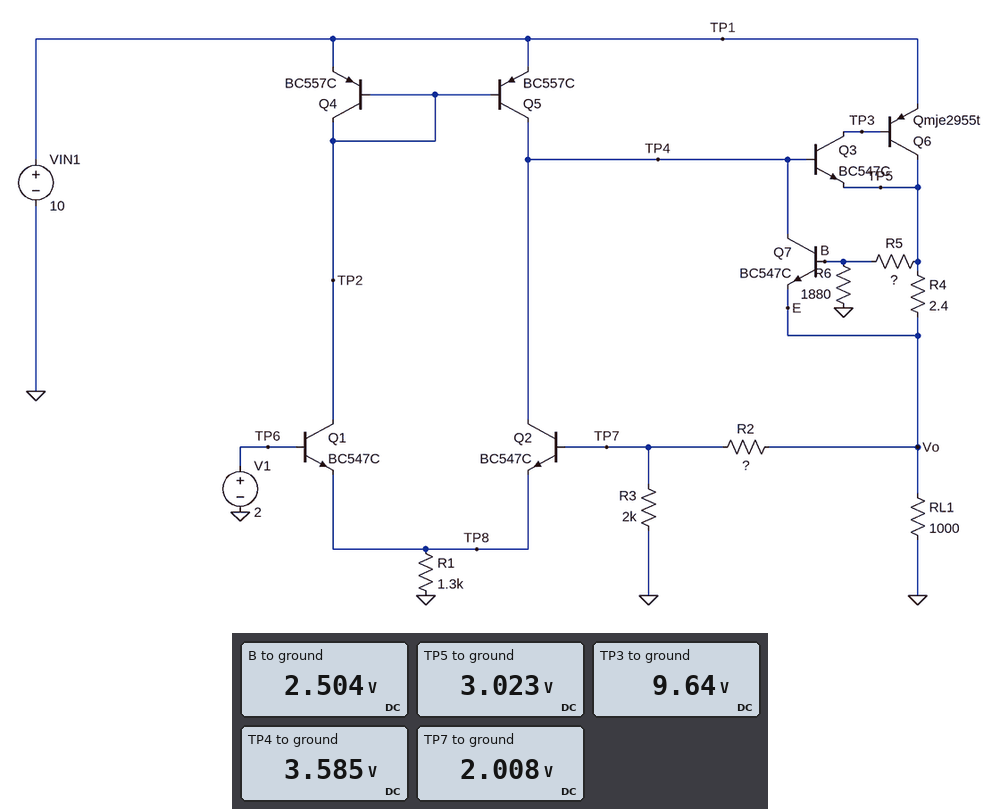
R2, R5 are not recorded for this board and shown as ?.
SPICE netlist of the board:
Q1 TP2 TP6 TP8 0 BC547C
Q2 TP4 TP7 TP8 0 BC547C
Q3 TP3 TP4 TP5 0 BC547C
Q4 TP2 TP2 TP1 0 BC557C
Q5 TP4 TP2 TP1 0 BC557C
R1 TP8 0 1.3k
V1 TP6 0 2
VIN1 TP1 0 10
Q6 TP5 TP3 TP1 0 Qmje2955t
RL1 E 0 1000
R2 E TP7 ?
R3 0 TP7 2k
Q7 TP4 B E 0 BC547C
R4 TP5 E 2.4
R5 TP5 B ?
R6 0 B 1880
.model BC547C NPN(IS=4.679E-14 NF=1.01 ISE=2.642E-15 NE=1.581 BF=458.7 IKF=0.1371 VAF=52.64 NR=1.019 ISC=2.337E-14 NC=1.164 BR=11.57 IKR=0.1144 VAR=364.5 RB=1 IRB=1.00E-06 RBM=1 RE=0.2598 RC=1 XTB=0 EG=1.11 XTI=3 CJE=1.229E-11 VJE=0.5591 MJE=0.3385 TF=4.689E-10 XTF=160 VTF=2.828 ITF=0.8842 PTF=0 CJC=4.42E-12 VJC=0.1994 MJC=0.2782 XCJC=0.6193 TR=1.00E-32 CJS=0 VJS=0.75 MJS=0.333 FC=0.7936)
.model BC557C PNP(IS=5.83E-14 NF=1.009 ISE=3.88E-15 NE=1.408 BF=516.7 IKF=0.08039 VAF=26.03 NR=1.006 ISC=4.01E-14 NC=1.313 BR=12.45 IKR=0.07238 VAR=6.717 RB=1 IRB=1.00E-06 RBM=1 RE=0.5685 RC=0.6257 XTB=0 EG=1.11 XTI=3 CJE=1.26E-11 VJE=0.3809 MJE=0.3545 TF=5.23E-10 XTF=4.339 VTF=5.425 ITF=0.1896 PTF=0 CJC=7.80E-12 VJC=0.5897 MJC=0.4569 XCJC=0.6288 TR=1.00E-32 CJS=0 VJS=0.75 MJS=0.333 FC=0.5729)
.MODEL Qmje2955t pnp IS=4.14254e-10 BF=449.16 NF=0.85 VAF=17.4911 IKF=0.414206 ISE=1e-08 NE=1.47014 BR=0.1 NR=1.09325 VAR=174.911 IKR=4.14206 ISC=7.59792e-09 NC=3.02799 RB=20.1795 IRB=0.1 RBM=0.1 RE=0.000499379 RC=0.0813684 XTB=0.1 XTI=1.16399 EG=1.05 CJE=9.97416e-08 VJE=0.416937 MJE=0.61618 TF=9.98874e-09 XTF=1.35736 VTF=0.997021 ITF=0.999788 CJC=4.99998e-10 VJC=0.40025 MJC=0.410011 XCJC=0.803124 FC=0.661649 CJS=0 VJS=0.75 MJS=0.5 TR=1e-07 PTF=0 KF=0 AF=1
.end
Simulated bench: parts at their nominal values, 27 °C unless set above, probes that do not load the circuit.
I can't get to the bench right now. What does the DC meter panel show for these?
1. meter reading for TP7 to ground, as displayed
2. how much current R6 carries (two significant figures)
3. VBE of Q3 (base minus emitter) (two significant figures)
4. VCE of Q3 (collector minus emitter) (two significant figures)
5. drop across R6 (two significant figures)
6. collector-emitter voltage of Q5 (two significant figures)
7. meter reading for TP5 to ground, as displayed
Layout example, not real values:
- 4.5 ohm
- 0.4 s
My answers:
- 2.008 V
- 1.3 mA
- 560 mV
- 6.6 V
- 2.5 V
- -6.4 V
- 3.023 V
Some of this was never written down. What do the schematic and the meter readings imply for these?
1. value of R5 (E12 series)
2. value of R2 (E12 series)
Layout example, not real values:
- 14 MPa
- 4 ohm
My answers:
- 390 Ω
- 1 kΩ
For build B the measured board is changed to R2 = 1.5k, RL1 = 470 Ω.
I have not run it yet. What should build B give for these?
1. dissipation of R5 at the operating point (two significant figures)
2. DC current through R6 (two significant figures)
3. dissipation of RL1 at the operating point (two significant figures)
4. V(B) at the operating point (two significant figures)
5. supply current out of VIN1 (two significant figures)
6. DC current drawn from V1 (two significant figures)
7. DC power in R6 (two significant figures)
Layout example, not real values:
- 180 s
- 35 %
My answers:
- 950 µW
- 1.6 mA
- 26 mW
- 2.9 V
- 11 mA
- 940 nA
- 4.6 mW
